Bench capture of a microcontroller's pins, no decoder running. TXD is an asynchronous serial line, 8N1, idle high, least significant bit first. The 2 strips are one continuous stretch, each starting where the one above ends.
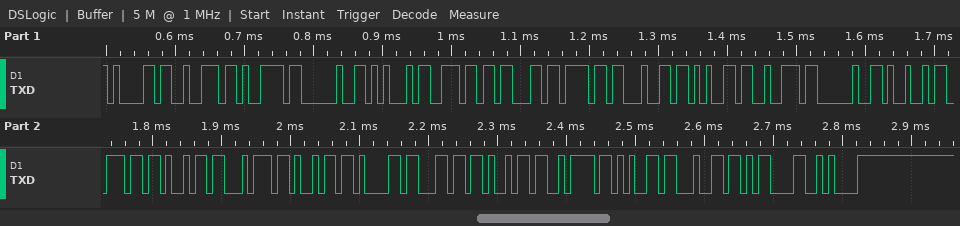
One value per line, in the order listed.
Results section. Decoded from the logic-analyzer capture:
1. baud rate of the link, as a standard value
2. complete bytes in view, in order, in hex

115200 baud
61 72 79 20 45 6E 63 6F 64 65 72 20 49 6E 69 74 69 61 6C 69 7A 65 64 0D 0A
